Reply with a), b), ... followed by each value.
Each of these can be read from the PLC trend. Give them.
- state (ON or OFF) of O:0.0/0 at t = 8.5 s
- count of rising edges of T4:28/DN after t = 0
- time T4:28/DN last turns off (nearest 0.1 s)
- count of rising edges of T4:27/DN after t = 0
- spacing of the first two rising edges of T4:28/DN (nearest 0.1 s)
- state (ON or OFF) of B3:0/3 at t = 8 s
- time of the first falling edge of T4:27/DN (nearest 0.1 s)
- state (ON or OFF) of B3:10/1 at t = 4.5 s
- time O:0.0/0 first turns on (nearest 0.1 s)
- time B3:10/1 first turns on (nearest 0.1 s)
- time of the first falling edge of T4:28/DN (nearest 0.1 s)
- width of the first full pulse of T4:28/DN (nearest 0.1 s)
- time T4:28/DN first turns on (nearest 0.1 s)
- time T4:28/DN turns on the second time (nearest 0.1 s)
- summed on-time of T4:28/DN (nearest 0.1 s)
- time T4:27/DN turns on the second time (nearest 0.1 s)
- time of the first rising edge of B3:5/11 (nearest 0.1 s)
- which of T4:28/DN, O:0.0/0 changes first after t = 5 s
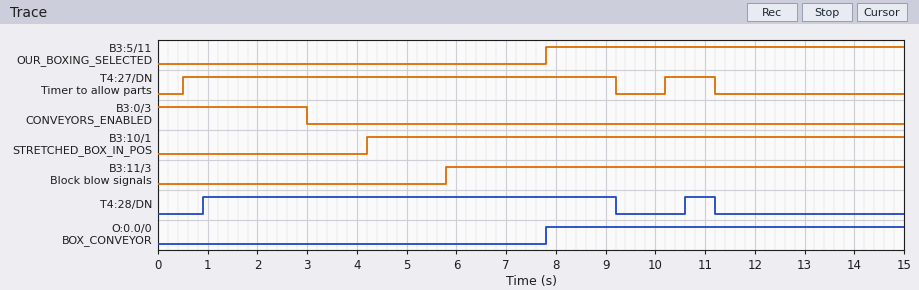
a) ON
b) 2
c) 11.2 s
d) 2
e) 9.7 s
f) OFF
g) 9.2 s
h) ON
i) 7.8 s
j) 4.2 s
k) 9.2 s
l) 8.3 s
m) 0.9 s
n) 10.6 s
o) 8.9 s
p) 10.2 s
q) 7.8 s
r) O:0.0/0
